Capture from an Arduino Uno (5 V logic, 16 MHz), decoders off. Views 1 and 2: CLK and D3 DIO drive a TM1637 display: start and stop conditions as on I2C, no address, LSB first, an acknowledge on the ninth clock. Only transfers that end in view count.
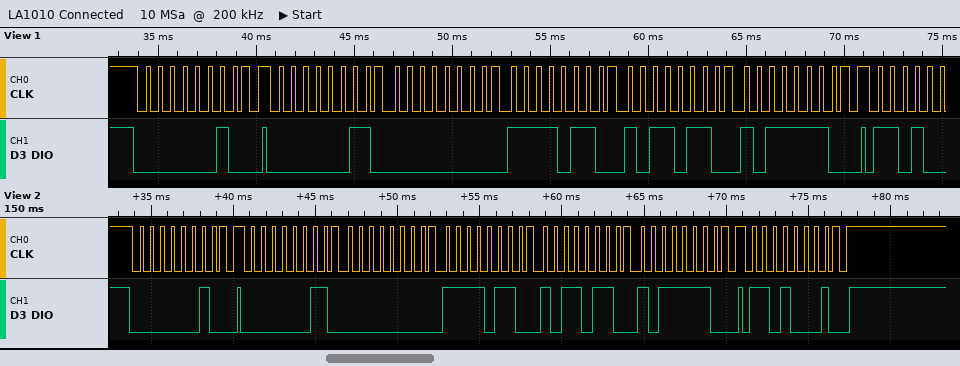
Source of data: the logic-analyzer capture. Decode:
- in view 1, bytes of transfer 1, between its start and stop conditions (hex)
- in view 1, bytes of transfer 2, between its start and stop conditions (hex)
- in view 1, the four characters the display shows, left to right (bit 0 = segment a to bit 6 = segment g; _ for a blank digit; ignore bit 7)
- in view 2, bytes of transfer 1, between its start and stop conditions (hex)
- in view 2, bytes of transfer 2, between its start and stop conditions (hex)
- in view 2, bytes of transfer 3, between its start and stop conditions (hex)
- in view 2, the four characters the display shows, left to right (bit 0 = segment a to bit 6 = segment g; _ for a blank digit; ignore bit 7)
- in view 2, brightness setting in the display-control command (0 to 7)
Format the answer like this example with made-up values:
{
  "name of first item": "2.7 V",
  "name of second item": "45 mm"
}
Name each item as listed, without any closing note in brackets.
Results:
{
  "in view 1, bytes of transfer 1, between its start and stop conditions": "40",
  "in view 1, bytes of transfer 2, between its start and stop conditions": "C0 00 6F 6D 7D",
  "in view 1, the four characters the display shows, left to right": "_956",
  "in view 2, bytes of transfer 1, between its start and stop conditions": "40",
  "in view 2, bytes of transfer 2, between its start and stop conditions": "C0 00 6F 6D 7D",
  "in view 2, bytes of transfer 3, between its start and stop conditions": "8B",
  "in view 2, the four characters the display shows, left to right": "_956",
  "in view 2, brightness setting in the display-control command": "3"
}
